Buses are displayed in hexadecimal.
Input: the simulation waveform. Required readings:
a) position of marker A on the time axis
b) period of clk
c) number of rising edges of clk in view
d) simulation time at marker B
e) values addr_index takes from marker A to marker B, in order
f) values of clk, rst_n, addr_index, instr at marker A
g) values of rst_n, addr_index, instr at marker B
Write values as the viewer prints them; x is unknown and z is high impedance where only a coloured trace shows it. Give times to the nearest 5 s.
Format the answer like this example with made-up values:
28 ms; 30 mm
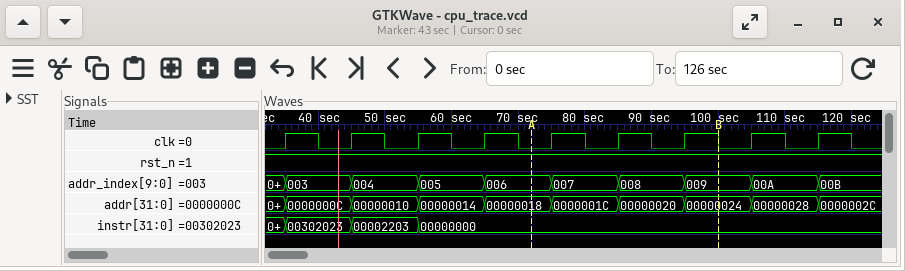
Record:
70 s; 10 s; 9; 100 s; 006, 007, 008, 009; clk=0, rst_n=1, addr_index=006, instr=00000000; rst_n=1, addr_index=009, instr=00000000
